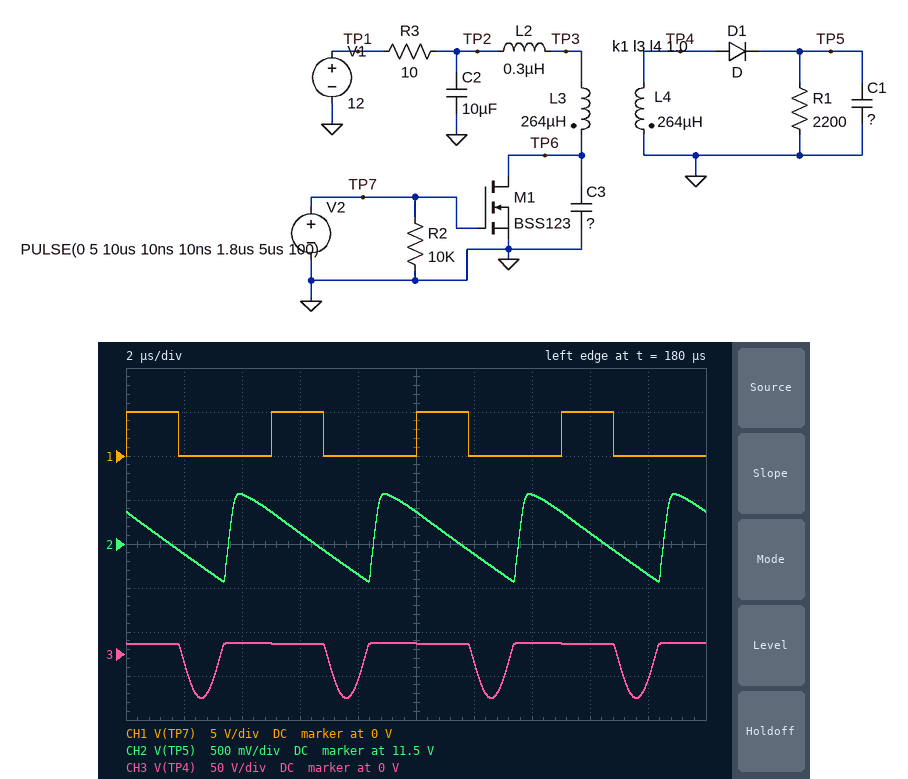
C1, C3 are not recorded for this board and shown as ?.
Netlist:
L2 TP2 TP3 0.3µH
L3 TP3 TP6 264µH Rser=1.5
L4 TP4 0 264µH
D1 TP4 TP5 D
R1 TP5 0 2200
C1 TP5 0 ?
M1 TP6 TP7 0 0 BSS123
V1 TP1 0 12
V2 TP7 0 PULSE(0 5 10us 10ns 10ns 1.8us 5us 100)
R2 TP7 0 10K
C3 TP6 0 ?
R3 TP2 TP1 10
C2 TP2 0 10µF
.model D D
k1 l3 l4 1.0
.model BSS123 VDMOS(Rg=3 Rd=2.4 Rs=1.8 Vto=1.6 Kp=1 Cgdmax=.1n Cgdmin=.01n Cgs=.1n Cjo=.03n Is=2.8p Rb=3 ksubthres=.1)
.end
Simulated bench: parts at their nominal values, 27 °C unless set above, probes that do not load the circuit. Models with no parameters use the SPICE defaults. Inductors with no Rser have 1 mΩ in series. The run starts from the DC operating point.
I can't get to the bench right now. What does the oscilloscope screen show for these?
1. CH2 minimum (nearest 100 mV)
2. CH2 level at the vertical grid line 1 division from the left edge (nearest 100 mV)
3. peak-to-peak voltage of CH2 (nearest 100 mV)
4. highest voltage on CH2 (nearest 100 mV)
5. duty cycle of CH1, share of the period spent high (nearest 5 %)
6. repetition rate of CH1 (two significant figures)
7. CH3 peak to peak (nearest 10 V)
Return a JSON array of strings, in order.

["11.1 V", "11.4 V", "1.0 V", "12.1 V", "35 %", "200 kHz", "60 V"]
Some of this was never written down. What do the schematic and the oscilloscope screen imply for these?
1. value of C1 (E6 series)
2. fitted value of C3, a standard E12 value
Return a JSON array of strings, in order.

["22 nF", "680 pF"]
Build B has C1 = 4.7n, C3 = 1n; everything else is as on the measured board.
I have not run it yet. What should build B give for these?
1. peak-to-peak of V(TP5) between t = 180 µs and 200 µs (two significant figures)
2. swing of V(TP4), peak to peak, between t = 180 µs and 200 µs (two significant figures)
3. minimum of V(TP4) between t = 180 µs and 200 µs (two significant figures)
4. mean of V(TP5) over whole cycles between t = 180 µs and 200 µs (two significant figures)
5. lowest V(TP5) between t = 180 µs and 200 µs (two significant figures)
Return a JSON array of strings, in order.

["3.2 V", "50 V", "-37 V", "11 V", "9.0 V"]
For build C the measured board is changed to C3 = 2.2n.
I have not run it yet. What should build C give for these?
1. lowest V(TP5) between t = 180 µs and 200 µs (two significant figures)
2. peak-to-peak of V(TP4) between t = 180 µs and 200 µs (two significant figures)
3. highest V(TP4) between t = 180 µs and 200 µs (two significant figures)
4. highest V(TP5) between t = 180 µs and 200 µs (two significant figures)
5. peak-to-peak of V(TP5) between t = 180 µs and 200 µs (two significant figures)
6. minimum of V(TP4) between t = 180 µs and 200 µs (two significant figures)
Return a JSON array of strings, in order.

["10 V", "29 V", "12 V", "11 V", "960 mV", "-17 V"]
